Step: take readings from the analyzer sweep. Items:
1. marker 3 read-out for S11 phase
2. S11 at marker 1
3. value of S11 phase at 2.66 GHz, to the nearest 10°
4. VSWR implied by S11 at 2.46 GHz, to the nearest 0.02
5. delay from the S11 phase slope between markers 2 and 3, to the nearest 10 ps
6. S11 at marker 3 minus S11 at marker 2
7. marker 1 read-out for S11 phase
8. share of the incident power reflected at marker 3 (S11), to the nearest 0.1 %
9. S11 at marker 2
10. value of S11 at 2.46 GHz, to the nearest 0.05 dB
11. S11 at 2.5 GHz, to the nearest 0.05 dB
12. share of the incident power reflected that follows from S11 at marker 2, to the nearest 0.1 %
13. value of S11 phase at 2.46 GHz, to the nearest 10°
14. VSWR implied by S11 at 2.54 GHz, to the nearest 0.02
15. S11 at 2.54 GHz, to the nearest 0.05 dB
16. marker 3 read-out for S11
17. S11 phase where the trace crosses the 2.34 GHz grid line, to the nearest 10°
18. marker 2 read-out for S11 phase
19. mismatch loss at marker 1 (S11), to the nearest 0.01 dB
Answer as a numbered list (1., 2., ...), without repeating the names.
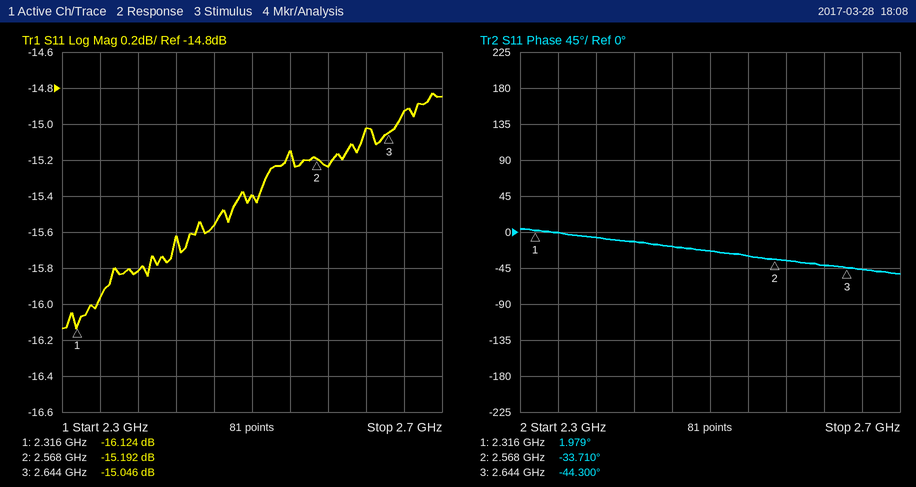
1. -44.300°
2. -16.124 dB
3. -50°
4. 1.40
5. 390 ps
6. 0.146 dB
7. 1.979°
8. 3.1 %
9. -15.192 dB
10. -15.55 dB
11. -15.40 dB
12. 3.0 %
13. -20°
14. 1.42
15. -15.15 dB
16. -15.046 dB
17. 0°
18. -33.710°
19. 0.11 dB
